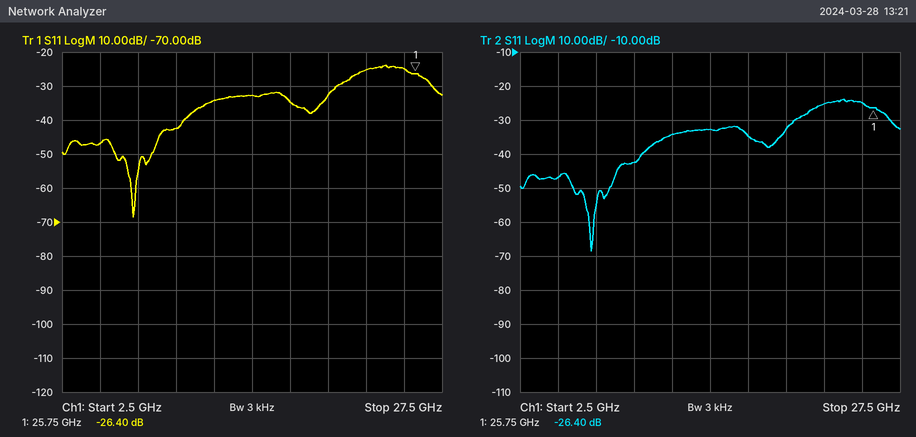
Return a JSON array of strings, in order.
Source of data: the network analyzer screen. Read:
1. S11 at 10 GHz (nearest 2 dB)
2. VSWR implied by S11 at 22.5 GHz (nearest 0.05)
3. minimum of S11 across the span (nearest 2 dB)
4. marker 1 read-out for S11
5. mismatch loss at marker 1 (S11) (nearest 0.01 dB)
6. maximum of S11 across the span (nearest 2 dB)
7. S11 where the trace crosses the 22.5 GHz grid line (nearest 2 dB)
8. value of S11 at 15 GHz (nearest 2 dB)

["-42 dB", "1.10", "-68 dB", "-26.40 dB", "0.01 dB", "-24 dB", "-26 dB", "-32 dB"]
